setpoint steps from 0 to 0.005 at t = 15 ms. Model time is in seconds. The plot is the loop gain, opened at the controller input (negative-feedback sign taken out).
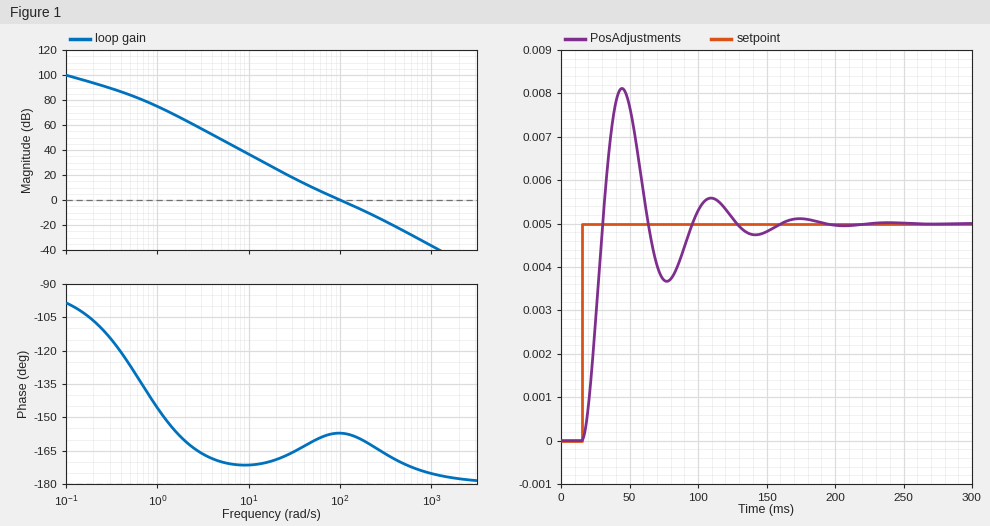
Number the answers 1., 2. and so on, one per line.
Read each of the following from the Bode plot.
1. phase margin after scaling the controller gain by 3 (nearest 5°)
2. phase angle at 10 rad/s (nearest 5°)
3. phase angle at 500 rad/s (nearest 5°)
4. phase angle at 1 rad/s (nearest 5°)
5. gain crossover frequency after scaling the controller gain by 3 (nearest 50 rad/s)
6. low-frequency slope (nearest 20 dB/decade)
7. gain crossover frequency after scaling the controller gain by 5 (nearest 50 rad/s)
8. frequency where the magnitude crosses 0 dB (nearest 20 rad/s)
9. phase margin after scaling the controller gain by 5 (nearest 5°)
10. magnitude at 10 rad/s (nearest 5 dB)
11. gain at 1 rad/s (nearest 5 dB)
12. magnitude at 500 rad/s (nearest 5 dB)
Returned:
1. 20°
2. -170°
3. -170°
4. -145°
5. 200 rad/s
6. -20 dB/decade
7. 250 rad/s
8. 100 rad/s
9. 15°
10. 35 dB
11. 75 dB
12. -25 dB
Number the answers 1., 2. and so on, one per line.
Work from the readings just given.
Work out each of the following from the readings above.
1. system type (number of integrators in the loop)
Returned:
1. 1
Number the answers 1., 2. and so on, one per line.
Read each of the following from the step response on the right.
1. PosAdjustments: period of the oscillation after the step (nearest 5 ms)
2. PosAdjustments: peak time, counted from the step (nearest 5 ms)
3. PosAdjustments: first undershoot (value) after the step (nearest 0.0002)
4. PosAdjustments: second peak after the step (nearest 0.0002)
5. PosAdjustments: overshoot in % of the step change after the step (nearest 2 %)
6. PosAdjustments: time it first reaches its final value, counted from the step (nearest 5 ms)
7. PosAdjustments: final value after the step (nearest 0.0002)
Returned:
1. 65 ms
2. 30 ms
3. 0.0036
4. 0.0056
5. 62 %
6. 15 ms
7. 0.0050
